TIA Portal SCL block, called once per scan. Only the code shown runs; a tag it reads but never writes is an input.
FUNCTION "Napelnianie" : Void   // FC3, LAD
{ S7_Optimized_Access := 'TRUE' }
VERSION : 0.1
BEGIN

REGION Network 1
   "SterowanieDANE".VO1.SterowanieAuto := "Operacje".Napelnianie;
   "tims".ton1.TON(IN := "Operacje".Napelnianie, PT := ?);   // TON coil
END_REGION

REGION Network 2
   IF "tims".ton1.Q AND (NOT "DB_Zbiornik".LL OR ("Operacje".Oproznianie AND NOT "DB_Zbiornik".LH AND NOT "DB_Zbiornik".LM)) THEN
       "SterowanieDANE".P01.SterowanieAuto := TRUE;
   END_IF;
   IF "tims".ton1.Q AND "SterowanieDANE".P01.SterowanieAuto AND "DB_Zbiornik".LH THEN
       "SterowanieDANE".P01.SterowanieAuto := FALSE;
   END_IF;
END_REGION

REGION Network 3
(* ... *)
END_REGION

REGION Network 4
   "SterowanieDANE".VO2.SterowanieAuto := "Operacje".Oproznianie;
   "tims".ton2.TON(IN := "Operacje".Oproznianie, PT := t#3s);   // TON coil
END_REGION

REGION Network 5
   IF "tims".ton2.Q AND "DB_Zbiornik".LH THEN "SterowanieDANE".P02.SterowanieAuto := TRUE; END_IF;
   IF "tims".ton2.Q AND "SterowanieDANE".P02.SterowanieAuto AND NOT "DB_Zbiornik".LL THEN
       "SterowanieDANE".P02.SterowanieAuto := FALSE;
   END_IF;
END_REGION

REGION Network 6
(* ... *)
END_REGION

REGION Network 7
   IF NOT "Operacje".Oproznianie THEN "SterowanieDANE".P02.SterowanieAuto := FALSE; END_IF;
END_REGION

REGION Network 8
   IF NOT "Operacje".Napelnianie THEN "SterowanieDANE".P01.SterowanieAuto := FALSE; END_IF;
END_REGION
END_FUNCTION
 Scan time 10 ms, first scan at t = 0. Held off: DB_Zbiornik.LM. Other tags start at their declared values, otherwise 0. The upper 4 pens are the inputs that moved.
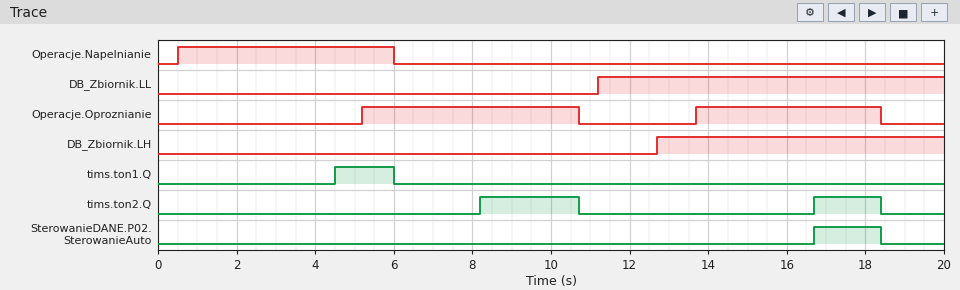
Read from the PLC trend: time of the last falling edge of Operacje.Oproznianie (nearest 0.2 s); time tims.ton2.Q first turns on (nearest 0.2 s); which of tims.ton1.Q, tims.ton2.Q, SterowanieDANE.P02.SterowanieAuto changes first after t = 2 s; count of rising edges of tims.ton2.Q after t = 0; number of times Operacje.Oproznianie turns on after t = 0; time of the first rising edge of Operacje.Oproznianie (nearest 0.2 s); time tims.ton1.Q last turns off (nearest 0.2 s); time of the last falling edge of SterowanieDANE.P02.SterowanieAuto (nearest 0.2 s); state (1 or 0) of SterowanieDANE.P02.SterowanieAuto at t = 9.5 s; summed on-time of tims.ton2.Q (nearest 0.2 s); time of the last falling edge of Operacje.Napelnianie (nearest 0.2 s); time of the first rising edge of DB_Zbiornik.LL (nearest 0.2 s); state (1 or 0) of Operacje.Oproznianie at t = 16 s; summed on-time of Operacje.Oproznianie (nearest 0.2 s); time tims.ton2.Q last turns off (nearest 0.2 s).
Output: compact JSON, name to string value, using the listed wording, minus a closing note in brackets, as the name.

{"time of the last falling edge of Operacje.Oproznianie": "18.4 s", "time tims.ton2.Q first turns on": "8.2 s", "which of tims.ton1.Q, tims.ton2.Q, SterowanieDANE.P02.SterowanieAuto changes first after t = 2 s": "tims.ton1.Q", "count of rising edges of tims.ton2.Q after t = 0": "2", "number of times Operacje.Oproznianie turns on after t = 0": "2", "time of the first rising edge of Operacje.Oproznianie": "5.2 s", "time tims.ton1.Q last turns off": "6.0 s", "time of the last falling edge of SterowanieDANE.P02.SterowanieAuto": "18.4 s", "state (1 or 0) of SterowanieDANE.P02.SterowanieAuto at t = 9.5 s": "0", "summed on-time of tims.ton2.Q": "4.2 s", "time of the last falling edge of Operacje.Napelnianie": "6.0 s", "time of the first rising edge of DB_Zbiornik.LL": "11.2 s", "state (1 or 0) of Operacje.Oproznianie at t = 16 s": "1", "summed on-time of Operacje.Oproznianie": "10.2 s", "time tims.ton2.Q last turns off": "18.4 s"}
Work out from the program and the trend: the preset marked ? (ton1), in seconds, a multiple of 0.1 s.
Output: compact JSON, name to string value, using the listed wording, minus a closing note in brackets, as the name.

{"the preset marked ? (ton1), in seconds, a multiple of 0.1 s": "4.0 s"}
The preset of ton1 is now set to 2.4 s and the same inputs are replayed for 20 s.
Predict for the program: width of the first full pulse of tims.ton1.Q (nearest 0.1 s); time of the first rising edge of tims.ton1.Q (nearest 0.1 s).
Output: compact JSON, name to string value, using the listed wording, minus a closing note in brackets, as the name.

{"width of the first full pulse of tims.ton1.Q": "3.1 s", "time of the first rising edge of tims.ton1.Q": "2.9 s"}
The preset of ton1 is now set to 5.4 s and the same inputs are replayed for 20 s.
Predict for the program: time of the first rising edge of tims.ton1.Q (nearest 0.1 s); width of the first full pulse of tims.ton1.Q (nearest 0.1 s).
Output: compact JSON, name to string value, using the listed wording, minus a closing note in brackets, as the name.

{"time of the first rising edge of tims.ton1.Q": "5.9 s", "width of the first full pulse of tims.ton1.Q": "0.1 s"}
